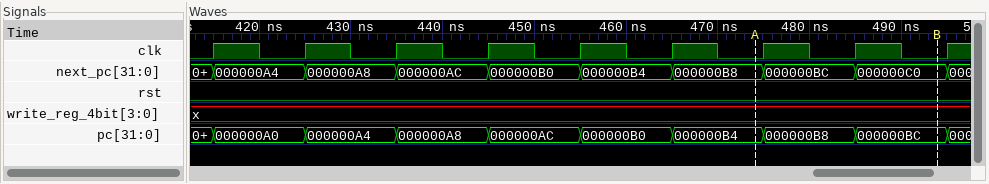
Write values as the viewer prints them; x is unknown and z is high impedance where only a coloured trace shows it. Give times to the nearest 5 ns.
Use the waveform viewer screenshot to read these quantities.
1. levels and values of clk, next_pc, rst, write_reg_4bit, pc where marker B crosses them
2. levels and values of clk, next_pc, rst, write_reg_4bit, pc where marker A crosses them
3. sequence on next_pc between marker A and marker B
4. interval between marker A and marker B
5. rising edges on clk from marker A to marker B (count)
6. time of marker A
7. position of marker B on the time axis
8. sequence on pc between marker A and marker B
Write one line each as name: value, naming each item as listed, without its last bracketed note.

levels and values of clk, next_pc, rst, write_reg_4bit, pc where marker B crosses them: clk=0, next_pc=000000C0, rst=0, write_reg_4bit=x, pc=000000BC
levels and values of clk, next_pc, rst, write_reg_4bit, pc where marker A crosses them: clk=0, next_pc=000000B8, rst=0, write_reg_4bit=x, pc=000000B4
sequence on next_pc between marker A and marker B: 000000B8, 000000BC, 000000C0
interval between marker A and marker B: 20 ns
rising edges on clk from marker A to marker B: 2
time of marker A: 475 ns
position of marker B on the time axis: 495 ns
sequence on pc between marker A and marker B: 000000B4, 000000B8, 000000BC
